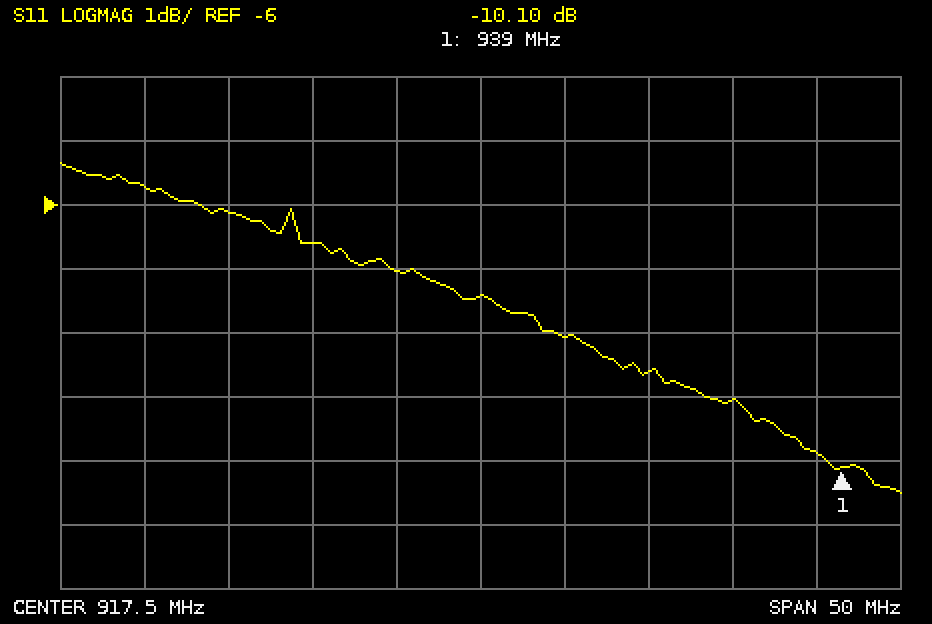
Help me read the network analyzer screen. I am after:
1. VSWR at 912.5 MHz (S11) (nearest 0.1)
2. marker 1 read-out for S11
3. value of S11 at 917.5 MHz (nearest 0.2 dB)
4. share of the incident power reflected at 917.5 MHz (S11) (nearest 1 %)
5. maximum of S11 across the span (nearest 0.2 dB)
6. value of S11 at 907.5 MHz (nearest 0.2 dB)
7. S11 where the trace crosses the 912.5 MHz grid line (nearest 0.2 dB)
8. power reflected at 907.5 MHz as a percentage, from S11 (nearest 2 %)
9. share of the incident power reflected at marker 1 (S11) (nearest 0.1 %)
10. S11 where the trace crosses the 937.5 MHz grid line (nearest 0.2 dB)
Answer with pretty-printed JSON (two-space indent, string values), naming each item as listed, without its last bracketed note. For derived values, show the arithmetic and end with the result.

{
  "VSWR at 912.5 MHz (S11)": "|Γ| = 10^(-7/20) = 0.4467; VSWR = (1 + 0.4467)/(1 − 0.4467) ≈ 2.6",
  "marker 1 read-out for S11": "-10.10 dB",
  "value of S11 at 917.5 MHz": "-7.4 dB",
  "share of the incident power reflected at 917.5 MHz (S11)": "10^(-7.4/10) ≈ 18 %",
  "maximum of S11 across the span": "-5.4 dB",
  "value of S11 at 907.5 MHz": "-6.6 dB",
  "S11 where the trace crosses the 912.5 MHz grid line": "-7.0 dB",
  "power reflected at 907.5 MHz as a percentage, from S11": "10^(-6.6/10) ≈ 22 %",
  "share of the incident power reflected at marker 1 (S11)": "10^(-10.1/10) ≈ 9.8 %",
  "S11 where the trace crosses the 937.5 MHz grid line": "-9.8 dB"
}
